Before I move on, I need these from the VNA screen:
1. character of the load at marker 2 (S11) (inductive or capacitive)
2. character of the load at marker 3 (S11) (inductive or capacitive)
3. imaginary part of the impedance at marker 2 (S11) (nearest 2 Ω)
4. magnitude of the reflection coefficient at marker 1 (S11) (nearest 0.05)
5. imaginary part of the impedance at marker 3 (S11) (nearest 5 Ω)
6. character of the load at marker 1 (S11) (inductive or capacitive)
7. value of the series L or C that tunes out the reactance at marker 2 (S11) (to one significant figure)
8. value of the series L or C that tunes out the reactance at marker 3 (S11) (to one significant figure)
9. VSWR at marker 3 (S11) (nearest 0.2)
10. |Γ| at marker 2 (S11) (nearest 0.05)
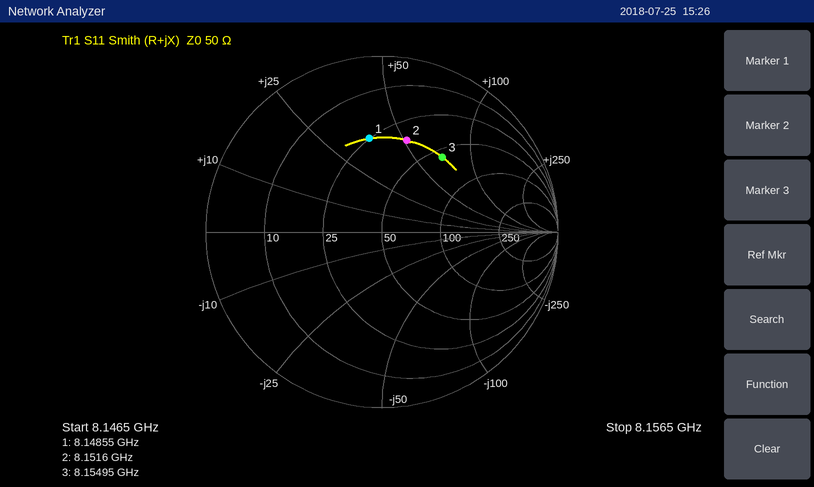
inductive
inductive
+52 Ω
0.55
+70 Ω
inductive
400 fF
300 fF
3.4
0.55
